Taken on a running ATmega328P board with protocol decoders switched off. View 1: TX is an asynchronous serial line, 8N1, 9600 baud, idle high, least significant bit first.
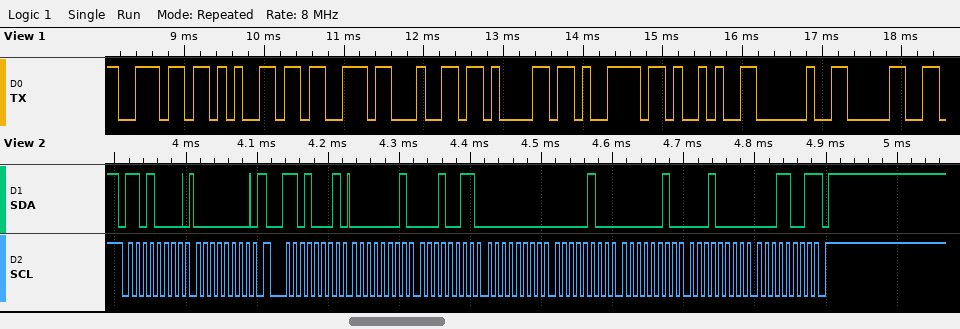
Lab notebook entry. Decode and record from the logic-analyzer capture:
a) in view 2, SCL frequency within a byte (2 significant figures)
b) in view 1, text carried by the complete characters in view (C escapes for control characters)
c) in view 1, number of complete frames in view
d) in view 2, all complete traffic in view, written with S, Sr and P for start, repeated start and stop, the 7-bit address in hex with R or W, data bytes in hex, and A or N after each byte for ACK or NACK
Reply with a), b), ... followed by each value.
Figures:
a) 100 kHz
b) "nesday) 0"
c) 9
d) S 68W A 00 A Sr 68R A 01 A 13 A 00 A 04 A 02 A 10 A 19 N P
